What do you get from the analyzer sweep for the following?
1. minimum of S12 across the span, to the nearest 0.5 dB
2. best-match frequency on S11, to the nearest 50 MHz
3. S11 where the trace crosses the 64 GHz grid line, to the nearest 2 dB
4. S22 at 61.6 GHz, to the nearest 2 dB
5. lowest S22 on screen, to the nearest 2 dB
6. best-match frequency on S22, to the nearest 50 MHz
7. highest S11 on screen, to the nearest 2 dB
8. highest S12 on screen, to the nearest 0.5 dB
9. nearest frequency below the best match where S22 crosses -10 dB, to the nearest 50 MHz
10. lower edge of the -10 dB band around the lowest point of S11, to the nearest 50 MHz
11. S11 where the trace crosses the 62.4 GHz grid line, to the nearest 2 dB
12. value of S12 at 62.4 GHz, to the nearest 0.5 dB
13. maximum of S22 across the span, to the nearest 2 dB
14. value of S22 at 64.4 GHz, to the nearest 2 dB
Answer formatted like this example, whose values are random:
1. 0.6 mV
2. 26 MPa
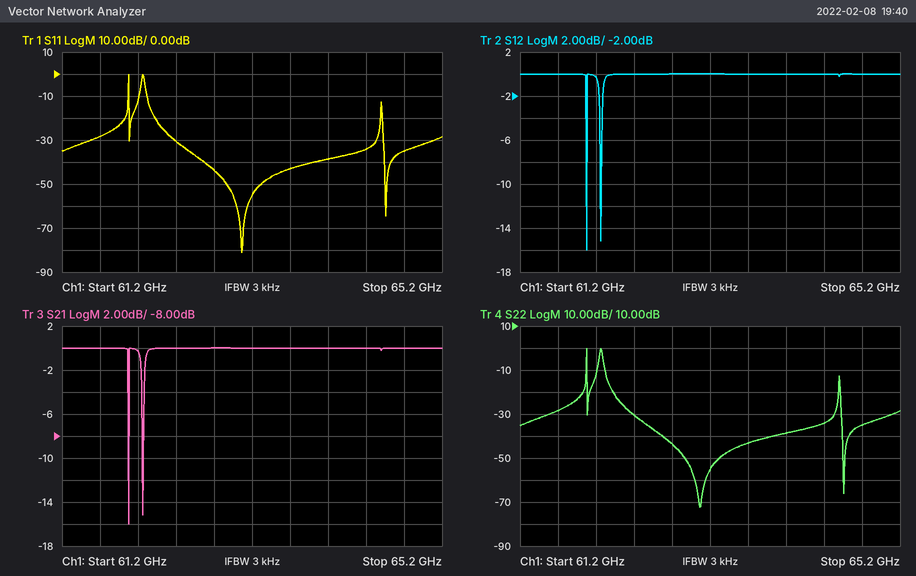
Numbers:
1. -16.0 dB
2. 63.10 GHz
3. -38 dB
4. -28 dB
5. -72 dB
6. 63.10 GHz
7. 0 dB
8. 0.0 dB
9. 62.10 GHz
10. 62.10 GHz
11. -30 dB
12. 0.0 dB
13. 0 dB
14. -34 dB
